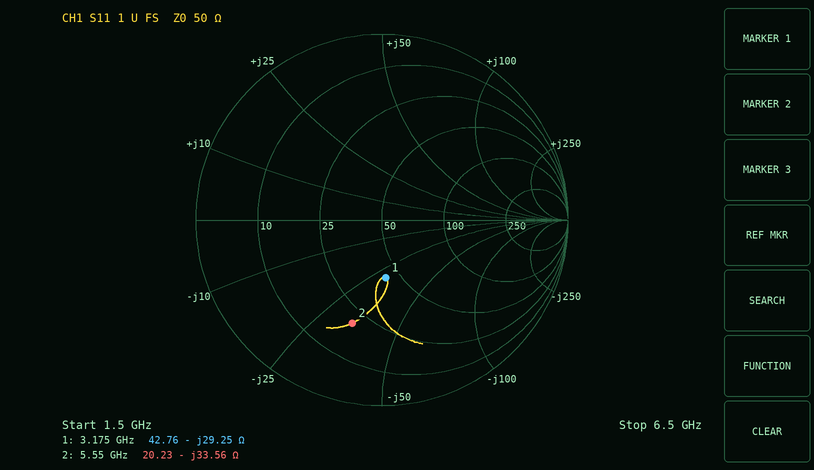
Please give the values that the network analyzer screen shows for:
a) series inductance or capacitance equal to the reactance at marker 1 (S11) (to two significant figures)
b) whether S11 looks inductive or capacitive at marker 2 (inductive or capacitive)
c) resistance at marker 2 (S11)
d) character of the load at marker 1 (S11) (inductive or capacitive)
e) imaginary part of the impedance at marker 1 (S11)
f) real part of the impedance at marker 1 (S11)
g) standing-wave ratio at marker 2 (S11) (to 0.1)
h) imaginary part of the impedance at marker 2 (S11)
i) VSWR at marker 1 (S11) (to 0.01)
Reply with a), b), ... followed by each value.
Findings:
a) 1.7 pF
b) capacitive
c) 20.23 Ω
d) capacitive
e) -29.25 Ω
f) 42.76 Ω
g) 3.7
h) -33.56 Ω
i) 1.90
